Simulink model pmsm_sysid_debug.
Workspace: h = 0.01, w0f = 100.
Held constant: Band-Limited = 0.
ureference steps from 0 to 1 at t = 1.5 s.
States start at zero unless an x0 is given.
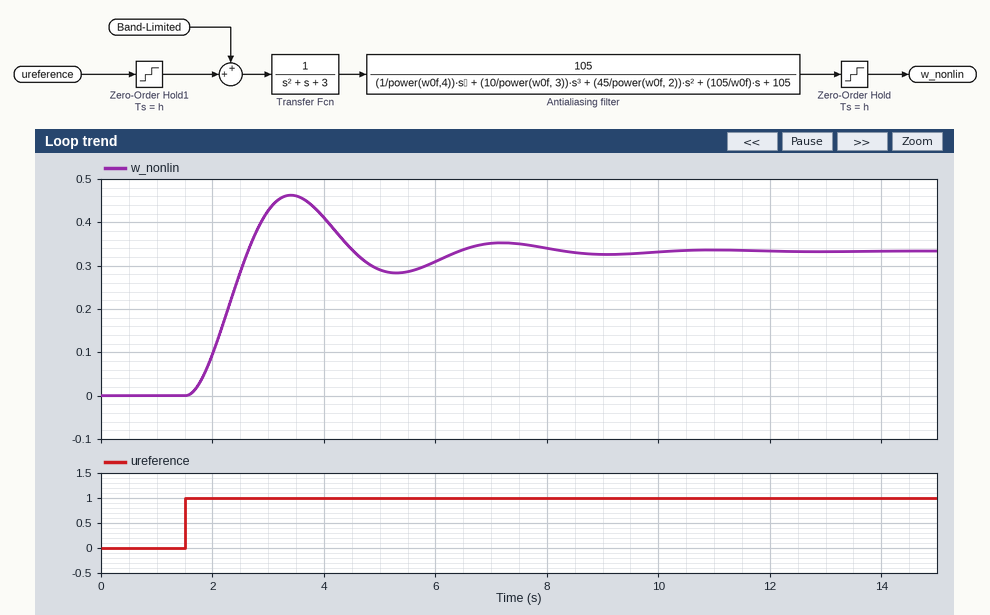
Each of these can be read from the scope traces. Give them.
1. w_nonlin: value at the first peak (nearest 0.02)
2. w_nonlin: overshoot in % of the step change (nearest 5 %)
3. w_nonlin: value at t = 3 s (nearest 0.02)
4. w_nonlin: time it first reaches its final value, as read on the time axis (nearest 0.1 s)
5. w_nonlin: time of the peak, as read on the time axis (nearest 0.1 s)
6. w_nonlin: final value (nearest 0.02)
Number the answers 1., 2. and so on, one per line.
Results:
1. 0.46
2. 40 %
3. 0.42
4. 2.6 s
5. 3.4 s
6. 0.34
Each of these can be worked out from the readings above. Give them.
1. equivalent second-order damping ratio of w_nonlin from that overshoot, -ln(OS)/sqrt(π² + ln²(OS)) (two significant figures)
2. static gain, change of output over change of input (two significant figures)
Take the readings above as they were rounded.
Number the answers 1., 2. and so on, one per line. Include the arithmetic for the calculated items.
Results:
1. ln(0.4) = -0.916; 0.916 / sqrt(9.870 + 0.840) = 0.28
2. (0.34 - 0) / (1 - 0) = 0.34
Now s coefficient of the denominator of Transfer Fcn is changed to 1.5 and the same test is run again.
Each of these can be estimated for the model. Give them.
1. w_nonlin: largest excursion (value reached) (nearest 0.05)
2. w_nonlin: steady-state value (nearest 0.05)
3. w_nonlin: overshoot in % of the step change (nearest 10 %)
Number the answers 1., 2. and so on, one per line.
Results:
1. 0.40
2. 0.35
3. 20 %
